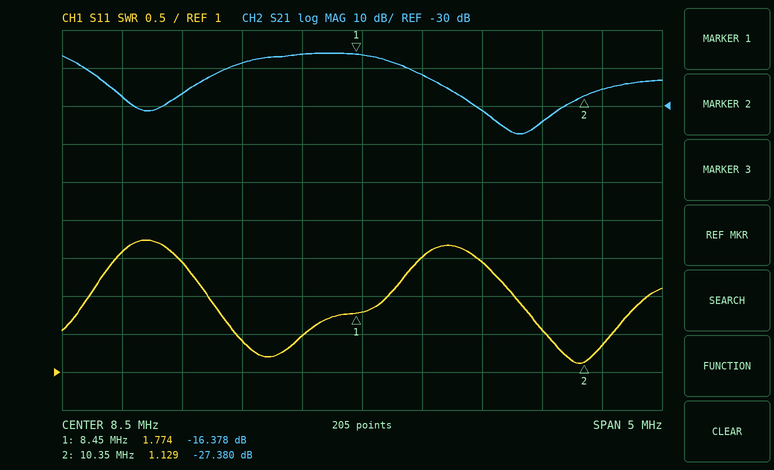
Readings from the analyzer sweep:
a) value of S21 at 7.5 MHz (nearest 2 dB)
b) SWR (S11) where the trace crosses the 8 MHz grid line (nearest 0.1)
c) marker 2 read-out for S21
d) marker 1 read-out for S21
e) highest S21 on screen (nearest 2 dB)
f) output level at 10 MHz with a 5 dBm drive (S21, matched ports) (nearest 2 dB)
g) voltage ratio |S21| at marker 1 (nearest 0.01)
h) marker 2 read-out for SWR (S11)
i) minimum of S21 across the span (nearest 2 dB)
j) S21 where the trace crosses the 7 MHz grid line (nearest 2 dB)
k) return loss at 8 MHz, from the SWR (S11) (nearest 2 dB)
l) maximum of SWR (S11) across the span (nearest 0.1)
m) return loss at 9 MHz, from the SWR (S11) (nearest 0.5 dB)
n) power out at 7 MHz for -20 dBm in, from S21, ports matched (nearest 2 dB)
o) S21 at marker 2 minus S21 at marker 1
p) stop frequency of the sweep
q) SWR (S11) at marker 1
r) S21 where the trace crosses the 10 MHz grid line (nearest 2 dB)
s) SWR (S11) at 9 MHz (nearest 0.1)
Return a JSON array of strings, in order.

["-18 dB", "1.5", "-27.380 dB", "-16.378 dB", "-16 dB", "-30 dBm", "0.15", "1.129", "-38 dB", "-26 dB", "14 dB", "2.7", "7.5 dB", "-46 dBm", "-11.002 dB", "11 MHz", "1.774", "-34 dB", "2.5"]
